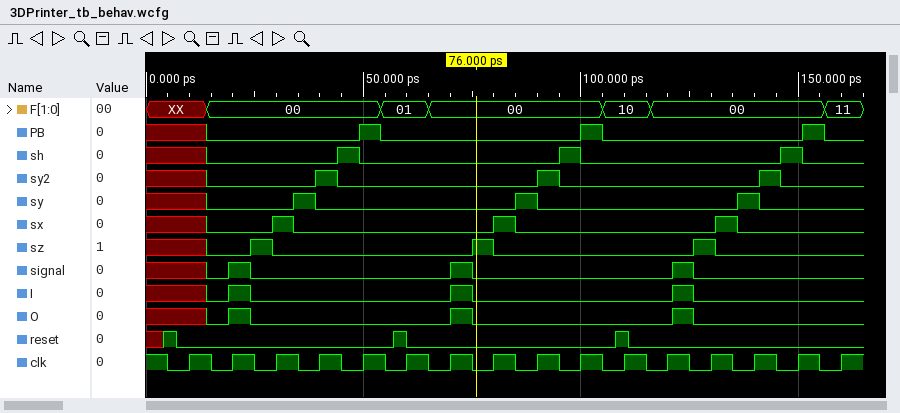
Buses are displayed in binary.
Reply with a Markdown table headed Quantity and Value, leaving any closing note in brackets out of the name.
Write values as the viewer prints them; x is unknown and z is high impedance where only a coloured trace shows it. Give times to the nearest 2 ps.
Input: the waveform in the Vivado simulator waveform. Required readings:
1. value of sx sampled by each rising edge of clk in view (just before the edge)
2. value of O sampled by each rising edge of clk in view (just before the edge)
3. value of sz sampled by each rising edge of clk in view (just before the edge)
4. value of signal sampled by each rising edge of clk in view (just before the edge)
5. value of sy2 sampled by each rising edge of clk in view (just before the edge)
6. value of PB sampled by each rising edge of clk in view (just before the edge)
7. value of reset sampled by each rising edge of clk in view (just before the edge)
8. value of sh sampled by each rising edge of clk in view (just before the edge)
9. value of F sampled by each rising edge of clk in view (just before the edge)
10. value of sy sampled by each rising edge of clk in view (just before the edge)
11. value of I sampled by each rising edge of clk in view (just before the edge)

| Quantity | Value |
|---|---|
| value of sx sampled by each rising edge of clk in view | x 0 1 0 0 0 0 0 0 0 0 0 0 0 0 0 |
| value of O sampled by each rising edge of clk in view | x 1 0 0 0 0 0 0 0 0 0 0 0 0 0 0 |
| value of sz sampled by each rising edge of clk in view | x 0 0 0 0 0 0 1 0 0 0 0 1 0 0 0 |
| value of signal sampled by each rising edge of clk in view | x 1 0 0 0 0 0 0 0 0 0 0 0 0 0 0 |
| value of sy2 sampled by each rising edge of clk in view | x 0 0 1 0 0 0 0 0 0 0 0 0 0 0 0 |
| value of PB sampled by each rising edge of clk in view | x 0 0 0 1 0 0 0 0 0 0 0 0 0 0 0 |
| value of reset sampled by each rising edge of clk in view | 0 0 0 0 0 1 0 0 0 0 1 0 0 0 0 0 |
| value of sh sampled by each rising edge of clk in view | x 0 0 0 0 0 0 0 0 1 0 0 0 0 1 0 |
| value of F sampled by each rising edge of clk in view | XX, 00, 00, 00, 00, 01, 00, 00, 00, 00, 10, 00, 00, 00, 00, 11 |
| value of sy sampled by each rising edge of clk in view | x 0 0 0 0 0 0 0 1 0 0 0 0 1 0 0 |
| value of I sampled by each rising edge of clk in view | x 1 0 0 0 0 0 0 0 0 0 0 0 0 0 0 |
